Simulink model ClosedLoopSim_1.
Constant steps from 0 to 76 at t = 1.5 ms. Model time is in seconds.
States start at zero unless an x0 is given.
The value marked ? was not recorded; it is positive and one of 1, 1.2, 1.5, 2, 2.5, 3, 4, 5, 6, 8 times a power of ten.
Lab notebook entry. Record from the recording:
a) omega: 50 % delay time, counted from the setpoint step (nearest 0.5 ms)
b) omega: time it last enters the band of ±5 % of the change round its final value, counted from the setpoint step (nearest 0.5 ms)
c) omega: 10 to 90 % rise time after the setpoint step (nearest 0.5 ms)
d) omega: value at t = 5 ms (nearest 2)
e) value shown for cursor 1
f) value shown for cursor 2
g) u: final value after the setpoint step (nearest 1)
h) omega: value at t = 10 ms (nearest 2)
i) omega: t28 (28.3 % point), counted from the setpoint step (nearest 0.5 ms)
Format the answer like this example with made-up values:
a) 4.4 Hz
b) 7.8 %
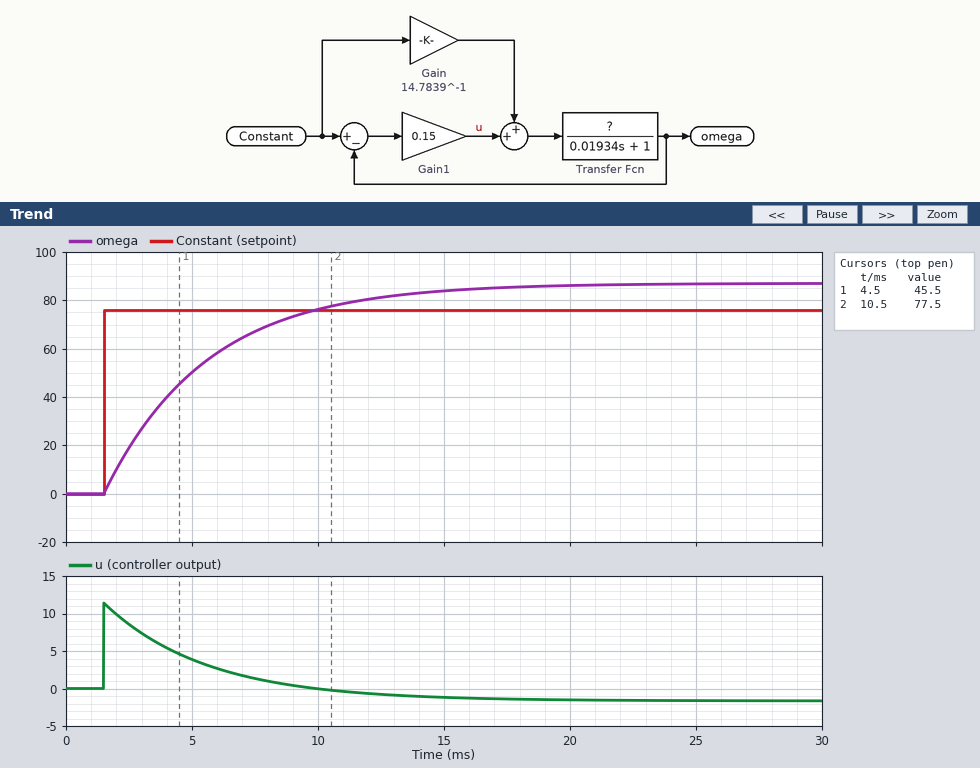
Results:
a) 3.0 ms
b) 12.0 ms
c) 9.0 ms
d) 50
e) 45.5
f) 77.5
g) -2
h) 76
i) 1.5 ms
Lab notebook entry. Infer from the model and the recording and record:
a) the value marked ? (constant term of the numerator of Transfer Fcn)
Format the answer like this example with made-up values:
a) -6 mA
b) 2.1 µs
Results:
a) 25
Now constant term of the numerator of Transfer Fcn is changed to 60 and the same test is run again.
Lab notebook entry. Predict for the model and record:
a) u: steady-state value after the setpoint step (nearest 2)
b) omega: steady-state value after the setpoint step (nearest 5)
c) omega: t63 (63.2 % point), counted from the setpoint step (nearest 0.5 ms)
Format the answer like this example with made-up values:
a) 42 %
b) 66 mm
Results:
a) -4
b) 100
c) 2.0 ms
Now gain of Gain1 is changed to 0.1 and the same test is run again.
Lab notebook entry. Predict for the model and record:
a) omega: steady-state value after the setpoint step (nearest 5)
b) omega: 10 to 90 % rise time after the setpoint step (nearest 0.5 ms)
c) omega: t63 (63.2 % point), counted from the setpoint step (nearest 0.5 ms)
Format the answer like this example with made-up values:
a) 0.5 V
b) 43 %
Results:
a) 90
b) 12.0 ms
c) 5.5 ms
